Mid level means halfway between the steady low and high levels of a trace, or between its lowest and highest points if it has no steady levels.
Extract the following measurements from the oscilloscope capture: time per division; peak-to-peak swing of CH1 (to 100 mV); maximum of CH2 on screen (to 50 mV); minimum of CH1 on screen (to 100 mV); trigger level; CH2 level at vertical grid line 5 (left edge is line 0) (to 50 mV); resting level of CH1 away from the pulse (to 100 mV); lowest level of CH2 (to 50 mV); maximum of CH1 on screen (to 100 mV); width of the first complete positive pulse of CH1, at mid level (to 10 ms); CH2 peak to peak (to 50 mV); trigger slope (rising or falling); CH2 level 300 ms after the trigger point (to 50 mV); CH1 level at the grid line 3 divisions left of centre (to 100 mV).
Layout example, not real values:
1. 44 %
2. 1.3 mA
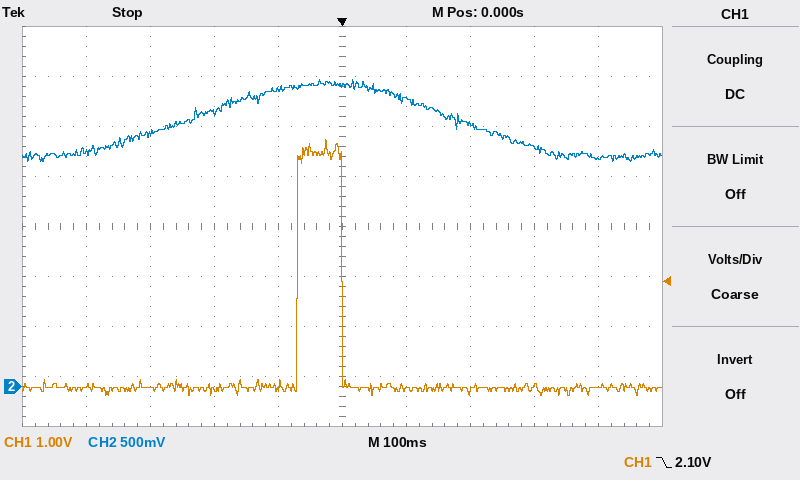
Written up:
1. 100 ms
2. 5.1 V
3. 3.05 V
4. -200 mV
5. 2.10 V
6. 3.00 V
7. 0.0 V
8. 2.25 V
9. 4.9 V
10. 70 ms
11. 800 mV
12. falling
13. 2.40 V
14. 0.0 V
